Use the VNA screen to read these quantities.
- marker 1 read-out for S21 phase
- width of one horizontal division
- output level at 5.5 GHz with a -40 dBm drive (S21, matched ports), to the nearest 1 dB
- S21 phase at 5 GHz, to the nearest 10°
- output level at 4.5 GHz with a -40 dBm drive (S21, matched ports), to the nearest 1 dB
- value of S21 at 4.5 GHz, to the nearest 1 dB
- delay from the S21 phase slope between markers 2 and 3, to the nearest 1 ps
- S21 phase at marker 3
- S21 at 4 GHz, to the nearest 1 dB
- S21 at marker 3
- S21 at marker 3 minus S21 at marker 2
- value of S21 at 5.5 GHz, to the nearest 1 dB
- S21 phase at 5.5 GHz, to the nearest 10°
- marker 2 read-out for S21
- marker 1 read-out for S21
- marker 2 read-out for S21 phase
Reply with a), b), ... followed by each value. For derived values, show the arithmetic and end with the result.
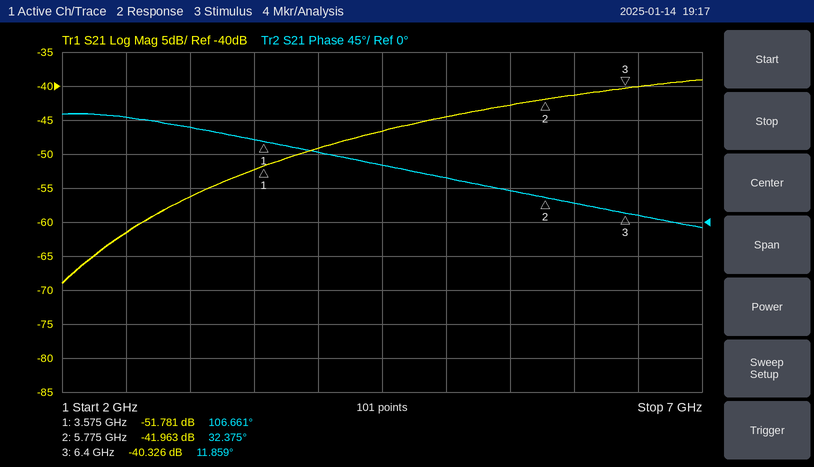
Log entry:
a) 106.661°
b) 500 MHz
c) -40 dBm + (-43 dB) = -83 dBm
d) 60°
e) -40 dBm + (-47 dB) = -87 dBm
f) -47 dB
g) −(11.859° − (32.375°))/(360° × 625 MHz) ≈ 91 ps
h) 11.859°
i) -49 dB
j) -40.326 dB
k) -40.326 − (-41.963) = 1.637 dB
l) -43 dB
m) 40°
n) -41.963 dB
o) -51.781 dB
p) 32.375°
